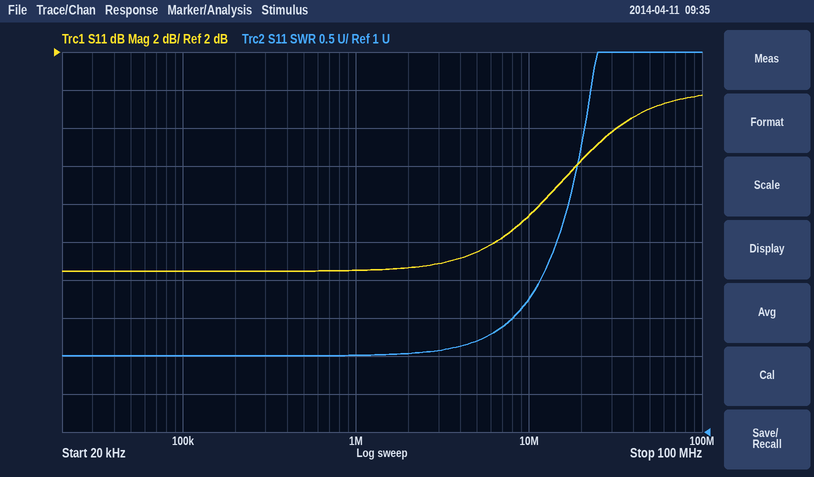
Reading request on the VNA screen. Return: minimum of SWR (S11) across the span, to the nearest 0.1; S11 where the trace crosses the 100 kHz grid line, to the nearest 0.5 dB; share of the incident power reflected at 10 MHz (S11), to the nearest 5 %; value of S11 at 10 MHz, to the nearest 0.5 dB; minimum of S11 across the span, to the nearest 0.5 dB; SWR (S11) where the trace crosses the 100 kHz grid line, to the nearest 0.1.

2.0
-9.5 dB
20 %
-6.5 dB
-9.5 dB
2.0
